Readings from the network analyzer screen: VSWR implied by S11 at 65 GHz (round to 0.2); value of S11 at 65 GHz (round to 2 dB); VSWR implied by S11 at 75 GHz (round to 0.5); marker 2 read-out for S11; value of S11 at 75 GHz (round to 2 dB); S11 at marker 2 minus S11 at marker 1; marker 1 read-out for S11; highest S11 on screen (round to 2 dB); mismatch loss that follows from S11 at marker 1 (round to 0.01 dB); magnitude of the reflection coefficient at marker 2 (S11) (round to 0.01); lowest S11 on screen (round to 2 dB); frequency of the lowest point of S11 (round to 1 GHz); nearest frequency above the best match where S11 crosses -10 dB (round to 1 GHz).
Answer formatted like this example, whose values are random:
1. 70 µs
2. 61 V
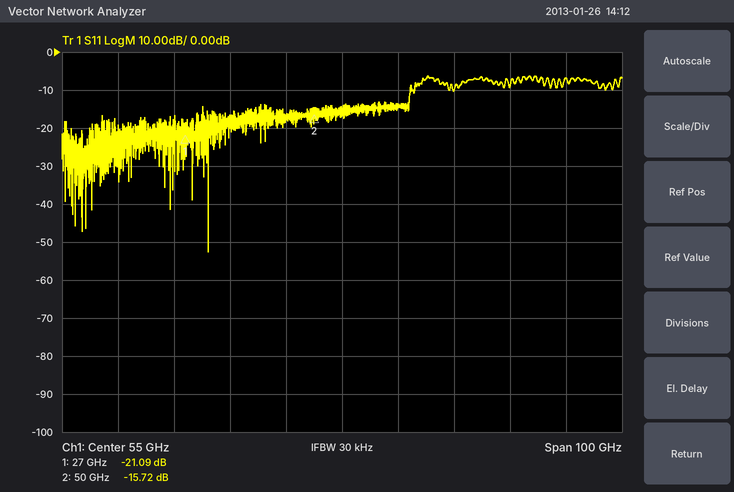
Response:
1. 1.4
2. -14 dB
3. 2.0
4. -15.72 dB
5. -10 dB
6. 5.37 dB
7. -21.09 dB
8. -6 dB
9. 0.03 dB
10. 0.16
11. -52 dB
12. 31 GHz
13. 67 GHz
